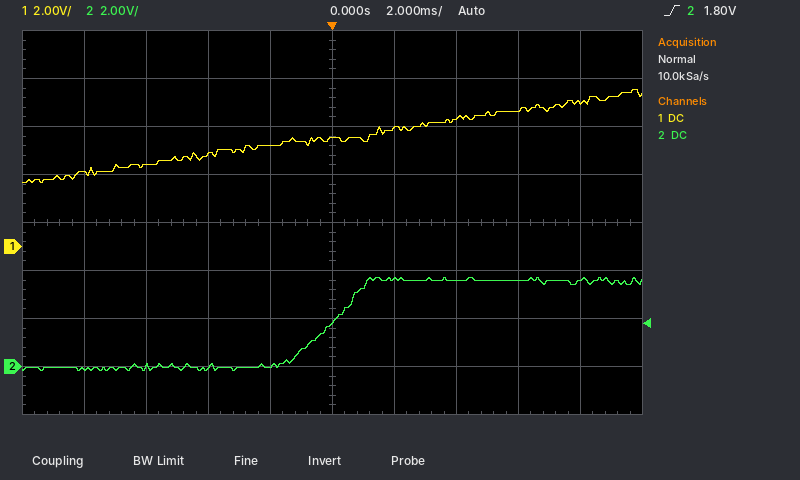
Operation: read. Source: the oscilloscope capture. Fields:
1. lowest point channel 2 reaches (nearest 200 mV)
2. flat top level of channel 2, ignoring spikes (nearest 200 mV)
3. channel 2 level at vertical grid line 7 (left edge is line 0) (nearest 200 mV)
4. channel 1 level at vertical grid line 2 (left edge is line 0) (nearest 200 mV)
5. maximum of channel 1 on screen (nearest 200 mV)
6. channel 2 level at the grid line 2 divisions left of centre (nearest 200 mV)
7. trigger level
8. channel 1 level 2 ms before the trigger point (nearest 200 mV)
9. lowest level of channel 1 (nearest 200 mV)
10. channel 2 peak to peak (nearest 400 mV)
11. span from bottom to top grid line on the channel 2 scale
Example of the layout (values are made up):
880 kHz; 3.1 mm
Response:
-200 mV; 3.6 V; 3.6 V; 3.4 V; 6.6 V; 0.0 V; 1.80 V; 4.2 V; 2.6 V; 4.0 V; 16 V
